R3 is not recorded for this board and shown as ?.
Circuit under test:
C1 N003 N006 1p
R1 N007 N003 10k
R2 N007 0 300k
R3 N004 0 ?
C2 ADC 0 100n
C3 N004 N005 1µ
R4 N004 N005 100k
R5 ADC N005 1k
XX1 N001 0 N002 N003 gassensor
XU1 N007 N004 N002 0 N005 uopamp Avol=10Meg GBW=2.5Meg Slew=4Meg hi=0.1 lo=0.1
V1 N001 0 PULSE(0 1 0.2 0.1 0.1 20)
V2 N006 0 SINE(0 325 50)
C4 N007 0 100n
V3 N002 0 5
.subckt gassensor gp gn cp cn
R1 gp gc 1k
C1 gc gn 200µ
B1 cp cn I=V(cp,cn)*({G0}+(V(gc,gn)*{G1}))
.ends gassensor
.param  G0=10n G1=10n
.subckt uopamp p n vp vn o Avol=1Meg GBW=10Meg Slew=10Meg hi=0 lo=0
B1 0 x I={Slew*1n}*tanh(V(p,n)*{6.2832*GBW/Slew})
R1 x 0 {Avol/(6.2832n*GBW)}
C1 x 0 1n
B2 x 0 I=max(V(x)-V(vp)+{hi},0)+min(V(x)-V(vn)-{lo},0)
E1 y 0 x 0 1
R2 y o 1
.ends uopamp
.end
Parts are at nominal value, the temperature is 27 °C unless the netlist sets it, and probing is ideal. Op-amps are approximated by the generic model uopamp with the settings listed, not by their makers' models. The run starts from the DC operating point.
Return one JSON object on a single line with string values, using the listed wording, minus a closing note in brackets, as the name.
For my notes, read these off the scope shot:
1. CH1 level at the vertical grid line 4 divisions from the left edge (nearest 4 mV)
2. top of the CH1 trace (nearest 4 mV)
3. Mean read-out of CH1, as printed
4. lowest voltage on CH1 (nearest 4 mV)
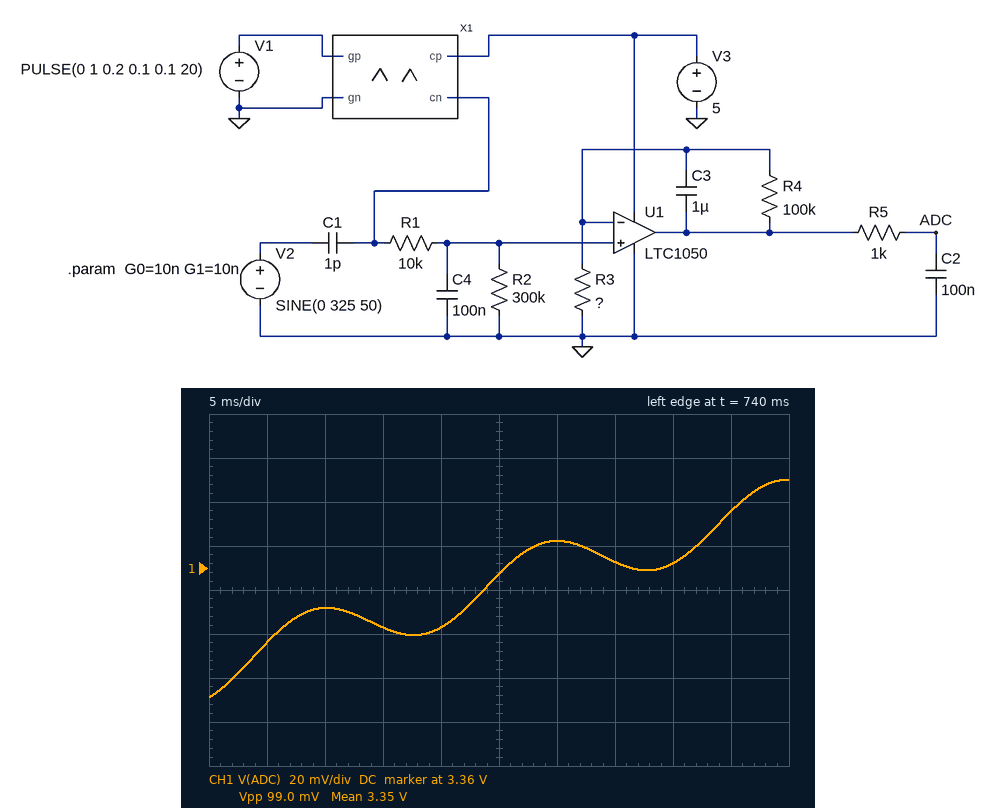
{"CH1 level at the vertical grid line 4 divisions from the left edge": "3.332 V", "top of the CH1 trace": "3.400 V", "Mean read-out of CH1, as printed": "3.35 V", "lowest voltage on CH1": "3.300 V"}
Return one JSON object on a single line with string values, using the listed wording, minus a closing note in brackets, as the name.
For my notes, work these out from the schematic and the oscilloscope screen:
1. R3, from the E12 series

{"R3, from the E12 series": "820 Ω"}
